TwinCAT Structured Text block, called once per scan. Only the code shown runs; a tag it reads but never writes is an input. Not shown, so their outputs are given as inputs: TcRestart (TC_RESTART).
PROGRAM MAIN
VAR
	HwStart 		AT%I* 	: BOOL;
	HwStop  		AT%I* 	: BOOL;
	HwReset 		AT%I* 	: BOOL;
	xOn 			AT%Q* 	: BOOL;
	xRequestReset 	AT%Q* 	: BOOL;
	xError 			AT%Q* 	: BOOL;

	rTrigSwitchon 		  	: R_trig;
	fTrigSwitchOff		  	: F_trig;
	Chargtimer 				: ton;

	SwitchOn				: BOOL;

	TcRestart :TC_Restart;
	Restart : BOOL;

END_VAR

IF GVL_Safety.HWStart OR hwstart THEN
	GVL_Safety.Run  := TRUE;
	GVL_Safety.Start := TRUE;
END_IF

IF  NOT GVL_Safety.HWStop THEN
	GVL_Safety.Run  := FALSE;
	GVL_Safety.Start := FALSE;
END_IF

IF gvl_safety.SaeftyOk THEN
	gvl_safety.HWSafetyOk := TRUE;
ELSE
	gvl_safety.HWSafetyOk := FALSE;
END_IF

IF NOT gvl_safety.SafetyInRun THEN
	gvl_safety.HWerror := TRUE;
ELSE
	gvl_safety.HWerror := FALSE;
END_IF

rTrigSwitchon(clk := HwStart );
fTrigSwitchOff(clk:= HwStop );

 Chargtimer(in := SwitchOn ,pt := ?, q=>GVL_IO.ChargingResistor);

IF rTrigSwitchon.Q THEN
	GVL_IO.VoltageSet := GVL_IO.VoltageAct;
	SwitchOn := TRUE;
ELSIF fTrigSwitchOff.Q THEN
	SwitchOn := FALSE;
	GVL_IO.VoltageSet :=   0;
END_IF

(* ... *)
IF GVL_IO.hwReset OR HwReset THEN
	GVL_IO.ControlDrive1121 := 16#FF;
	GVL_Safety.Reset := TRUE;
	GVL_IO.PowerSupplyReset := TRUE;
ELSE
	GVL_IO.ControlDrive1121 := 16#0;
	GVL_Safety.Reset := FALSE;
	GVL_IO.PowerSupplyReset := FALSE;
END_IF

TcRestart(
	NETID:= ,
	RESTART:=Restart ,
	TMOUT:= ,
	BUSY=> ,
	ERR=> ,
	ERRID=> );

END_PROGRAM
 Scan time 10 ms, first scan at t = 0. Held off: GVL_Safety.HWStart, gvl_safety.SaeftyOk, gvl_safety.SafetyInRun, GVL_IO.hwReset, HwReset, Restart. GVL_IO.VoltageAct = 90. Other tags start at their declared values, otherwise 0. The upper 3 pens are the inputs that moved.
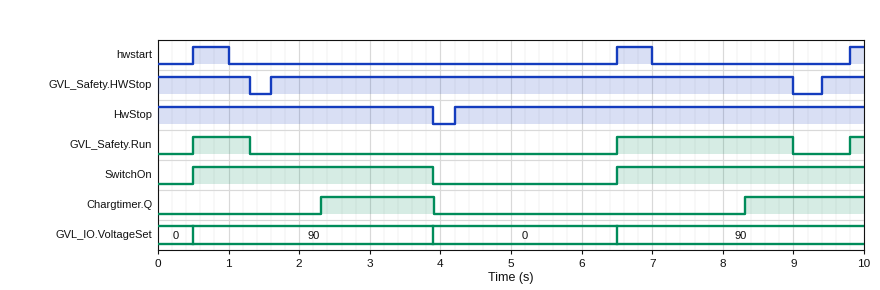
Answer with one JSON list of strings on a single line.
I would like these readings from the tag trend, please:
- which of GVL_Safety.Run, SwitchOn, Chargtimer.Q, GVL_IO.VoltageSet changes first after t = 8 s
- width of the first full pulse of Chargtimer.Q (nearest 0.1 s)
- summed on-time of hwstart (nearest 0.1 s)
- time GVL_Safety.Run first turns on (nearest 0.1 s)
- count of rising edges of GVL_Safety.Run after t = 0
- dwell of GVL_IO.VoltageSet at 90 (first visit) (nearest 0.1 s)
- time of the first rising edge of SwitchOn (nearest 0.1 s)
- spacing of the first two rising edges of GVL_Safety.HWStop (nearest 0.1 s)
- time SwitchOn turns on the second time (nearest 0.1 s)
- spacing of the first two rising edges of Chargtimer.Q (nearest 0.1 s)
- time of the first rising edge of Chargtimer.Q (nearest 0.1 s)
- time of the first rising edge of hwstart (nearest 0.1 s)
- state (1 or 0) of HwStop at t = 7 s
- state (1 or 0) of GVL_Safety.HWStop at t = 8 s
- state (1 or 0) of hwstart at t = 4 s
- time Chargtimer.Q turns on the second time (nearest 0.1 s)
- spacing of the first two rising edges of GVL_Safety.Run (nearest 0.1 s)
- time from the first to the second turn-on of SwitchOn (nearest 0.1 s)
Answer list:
["Chargtimer.Q", "1.6 s", "1.2 s", "0.5 s", "3", "3.4 s", "0.5 s", "7.8 s", "6.5 s", "6.0 s", "2.3 s", "0.5 s", "1", "1", "0", "8.3 s", "6.0 s", "6.0 s"]
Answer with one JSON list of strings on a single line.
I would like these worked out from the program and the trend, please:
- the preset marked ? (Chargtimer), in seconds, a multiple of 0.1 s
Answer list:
["1.8 s"]
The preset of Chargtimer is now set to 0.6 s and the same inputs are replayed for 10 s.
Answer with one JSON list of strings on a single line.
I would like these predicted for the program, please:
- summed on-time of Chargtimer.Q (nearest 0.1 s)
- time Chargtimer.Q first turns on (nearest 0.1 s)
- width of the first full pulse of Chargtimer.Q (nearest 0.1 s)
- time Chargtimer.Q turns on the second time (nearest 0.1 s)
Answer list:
["5.7 s", "1.1 s", "2.8 s", "7.1 s"]
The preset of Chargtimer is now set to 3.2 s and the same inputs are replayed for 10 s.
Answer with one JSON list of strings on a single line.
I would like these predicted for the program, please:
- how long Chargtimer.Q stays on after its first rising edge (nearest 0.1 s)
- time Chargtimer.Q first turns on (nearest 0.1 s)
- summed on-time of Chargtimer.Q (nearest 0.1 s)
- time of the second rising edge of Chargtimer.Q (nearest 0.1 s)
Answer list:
["0.2 s", "3.7 s", "0.5 s", "9.7 s"]
